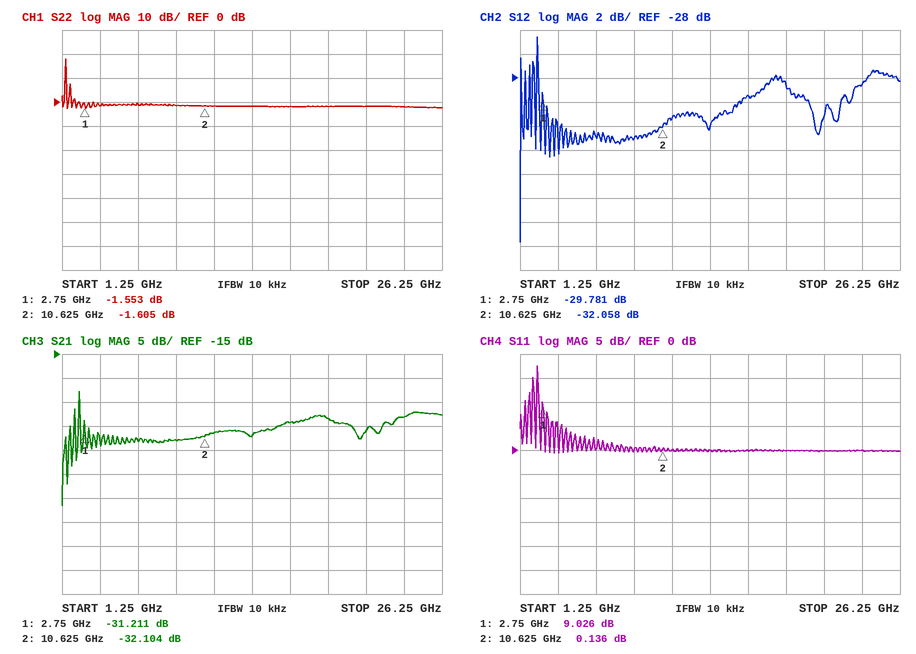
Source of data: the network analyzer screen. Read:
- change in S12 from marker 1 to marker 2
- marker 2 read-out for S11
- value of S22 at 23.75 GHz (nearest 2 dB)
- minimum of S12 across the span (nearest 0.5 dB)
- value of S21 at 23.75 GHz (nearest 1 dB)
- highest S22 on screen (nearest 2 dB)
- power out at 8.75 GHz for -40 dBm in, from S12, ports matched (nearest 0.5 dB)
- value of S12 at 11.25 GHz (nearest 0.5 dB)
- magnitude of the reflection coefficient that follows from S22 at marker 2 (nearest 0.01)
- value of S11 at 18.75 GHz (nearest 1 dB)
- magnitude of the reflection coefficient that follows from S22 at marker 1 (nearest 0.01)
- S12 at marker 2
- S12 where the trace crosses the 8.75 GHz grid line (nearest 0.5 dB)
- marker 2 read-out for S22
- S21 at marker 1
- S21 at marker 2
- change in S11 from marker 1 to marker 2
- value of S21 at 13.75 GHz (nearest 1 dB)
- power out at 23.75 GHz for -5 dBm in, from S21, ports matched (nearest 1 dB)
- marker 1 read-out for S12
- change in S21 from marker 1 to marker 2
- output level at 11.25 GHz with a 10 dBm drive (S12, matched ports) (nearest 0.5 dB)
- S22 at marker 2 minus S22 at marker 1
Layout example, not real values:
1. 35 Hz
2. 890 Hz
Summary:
1. -2.277 dB
2. 0.136 dB
3. -2 dB
4. -41.5 dB
5. -28 dB
6. 18 dB
7. -73.0 dBm
8. -31.5 dB
9. 0.83
10. 0 dB
11. 0.84
12. -32.058 dB
13. -33.0 dB
14. -1.605 dB
15. -31.211 dB
16. -32.104 dB
17. -8.890 dB
18. -32 dB
19. -33 dBm
20. -29.781 dB
21. -0.893 dB
22. -21.5 dBm
23. -0.052 dB
